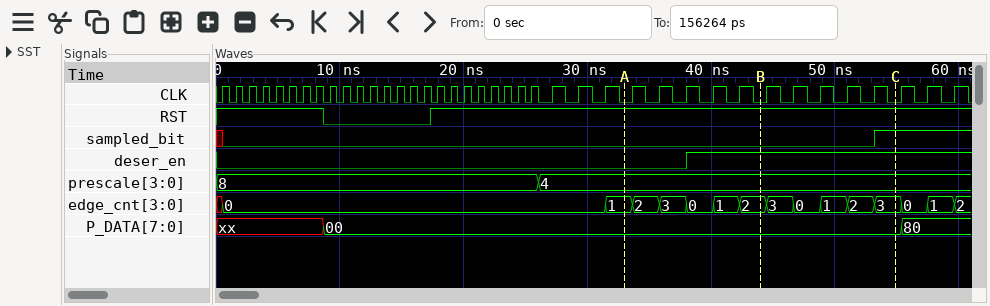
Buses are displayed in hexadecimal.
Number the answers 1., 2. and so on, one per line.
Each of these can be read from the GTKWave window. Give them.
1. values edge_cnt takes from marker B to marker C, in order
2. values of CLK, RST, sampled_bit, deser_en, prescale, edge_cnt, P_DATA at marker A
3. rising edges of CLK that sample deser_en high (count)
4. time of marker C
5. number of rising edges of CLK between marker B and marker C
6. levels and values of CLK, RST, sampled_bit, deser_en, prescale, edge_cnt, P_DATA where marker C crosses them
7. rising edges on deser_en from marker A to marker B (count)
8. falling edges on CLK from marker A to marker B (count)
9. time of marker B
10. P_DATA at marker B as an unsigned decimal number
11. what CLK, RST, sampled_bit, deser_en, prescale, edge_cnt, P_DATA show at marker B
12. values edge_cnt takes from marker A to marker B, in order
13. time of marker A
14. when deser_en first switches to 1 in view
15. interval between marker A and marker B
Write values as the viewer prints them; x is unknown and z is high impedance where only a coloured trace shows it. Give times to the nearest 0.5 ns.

1. 2, 3, 0, 1, 2, 3
2. CLK=0, RST=1, sampled_bit=0, deser_en=0, prescale=4, edge_cnt=1, P_DATA=00
3. 10
4. 55 ns
5. 5
6. CLK=0, RST=1, sampled_bit=1, deser_en=1, prescale=4, edge_cnt=3, P_DATA=00
7. 1
8. 5
9. 44 ns
10. 0
11. CLK=0, RST=1, sampled_bit=0, deser_en=1, prescale=4, edge_cnt=2, P_DATA=00
12. 1, 2, 3, 0, 1, 2
13. 33 ns
14. 38 ns
15. 11 ns
